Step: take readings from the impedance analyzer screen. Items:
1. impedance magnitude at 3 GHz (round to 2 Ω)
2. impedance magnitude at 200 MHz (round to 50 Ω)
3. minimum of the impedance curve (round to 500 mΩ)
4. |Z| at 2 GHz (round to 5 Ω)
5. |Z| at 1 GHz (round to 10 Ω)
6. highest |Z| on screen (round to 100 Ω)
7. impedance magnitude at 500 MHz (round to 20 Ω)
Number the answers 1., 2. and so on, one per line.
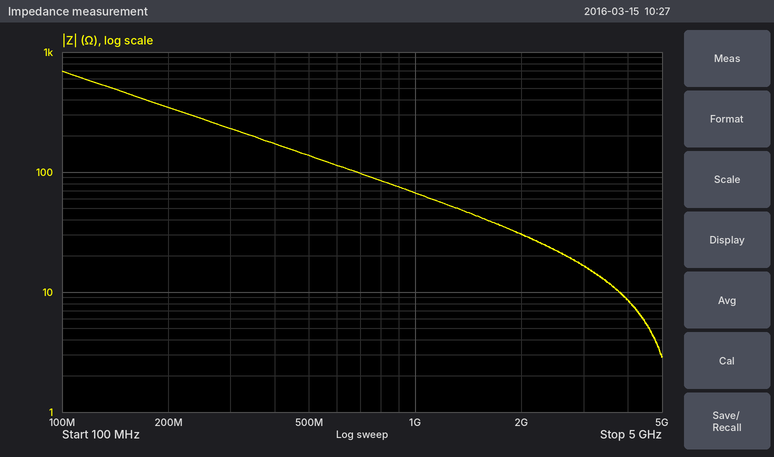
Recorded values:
1. 16 Ω
2. 350 Ω
3. 3.0 Ω
4. 30 Ω
5. 70 Ω
6. 700 Ω
7. 140 Ω
